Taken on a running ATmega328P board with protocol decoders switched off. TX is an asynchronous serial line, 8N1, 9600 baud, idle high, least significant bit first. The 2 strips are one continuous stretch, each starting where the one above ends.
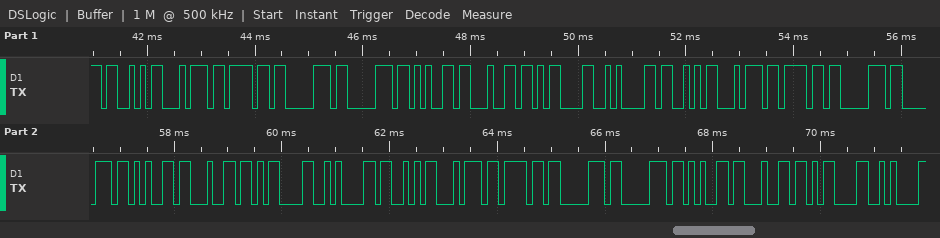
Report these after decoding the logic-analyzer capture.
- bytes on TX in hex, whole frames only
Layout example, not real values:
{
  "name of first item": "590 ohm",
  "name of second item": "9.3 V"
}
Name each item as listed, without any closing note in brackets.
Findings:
{
  "bytes on TX in hex, whole frames only": "53 74 6F 70 70 65 64 0D 0A 53 74 6F 70 70 65 64 0D 0A 53 74 6F 70 70 65 64 0D 0A"
}
